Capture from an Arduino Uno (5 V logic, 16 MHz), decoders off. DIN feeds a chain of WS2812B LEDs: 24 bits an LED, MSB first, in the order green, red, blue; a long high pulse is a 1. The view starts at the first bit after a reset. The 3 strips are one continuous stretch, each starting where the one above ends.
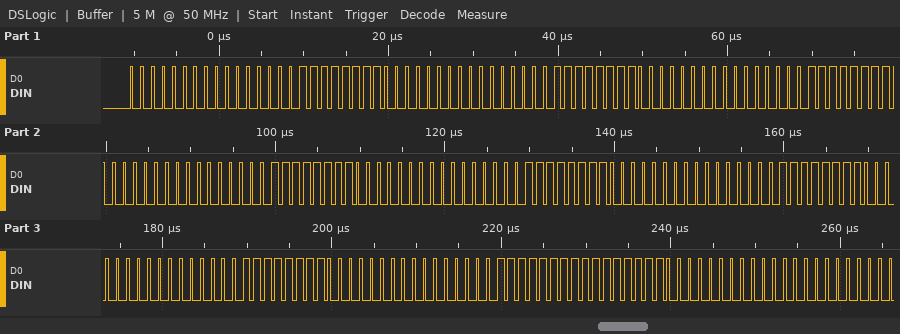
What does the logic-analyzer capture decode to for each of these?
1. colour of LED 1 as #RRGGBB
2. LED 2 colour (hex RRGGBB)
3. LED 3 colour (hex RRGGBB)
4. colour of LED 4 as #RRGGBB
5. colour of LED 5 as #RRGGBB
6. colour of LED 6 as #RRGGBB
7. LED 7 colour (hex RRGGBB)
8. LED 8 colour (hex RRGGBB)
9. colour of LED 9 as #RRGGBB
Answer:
#0000FF
#0000FF
#0000FF
#0000FF
#0000FF
#0000FF
#0000FF
#0000FF
#00FF00
